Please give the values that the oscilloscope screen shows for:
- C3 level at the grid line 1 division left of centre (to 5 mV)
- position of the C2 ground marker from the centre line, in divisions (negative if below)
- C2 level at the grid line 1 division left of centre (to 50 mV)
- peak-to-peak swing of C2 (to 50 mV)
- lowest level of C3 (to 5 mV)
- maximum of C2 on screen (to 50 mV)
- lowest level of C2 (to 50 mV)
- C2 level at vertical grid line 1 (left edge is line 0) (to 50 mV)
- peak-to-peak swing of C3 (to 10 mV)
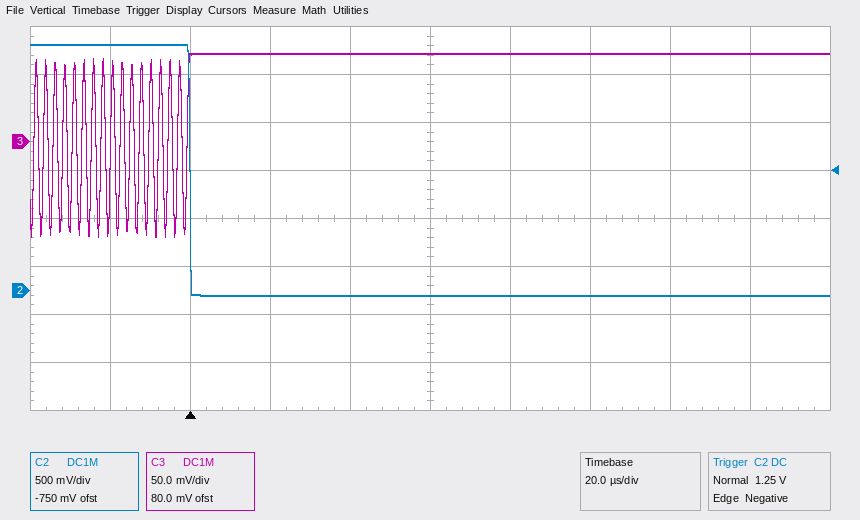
90 mV
-1.5 div
-50 mV
2.60 V
-100 mV
2.55 V
-50 mV
2.55 V
190 mV
